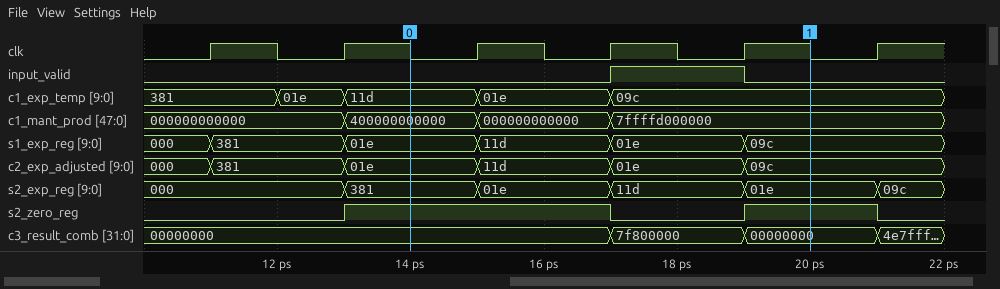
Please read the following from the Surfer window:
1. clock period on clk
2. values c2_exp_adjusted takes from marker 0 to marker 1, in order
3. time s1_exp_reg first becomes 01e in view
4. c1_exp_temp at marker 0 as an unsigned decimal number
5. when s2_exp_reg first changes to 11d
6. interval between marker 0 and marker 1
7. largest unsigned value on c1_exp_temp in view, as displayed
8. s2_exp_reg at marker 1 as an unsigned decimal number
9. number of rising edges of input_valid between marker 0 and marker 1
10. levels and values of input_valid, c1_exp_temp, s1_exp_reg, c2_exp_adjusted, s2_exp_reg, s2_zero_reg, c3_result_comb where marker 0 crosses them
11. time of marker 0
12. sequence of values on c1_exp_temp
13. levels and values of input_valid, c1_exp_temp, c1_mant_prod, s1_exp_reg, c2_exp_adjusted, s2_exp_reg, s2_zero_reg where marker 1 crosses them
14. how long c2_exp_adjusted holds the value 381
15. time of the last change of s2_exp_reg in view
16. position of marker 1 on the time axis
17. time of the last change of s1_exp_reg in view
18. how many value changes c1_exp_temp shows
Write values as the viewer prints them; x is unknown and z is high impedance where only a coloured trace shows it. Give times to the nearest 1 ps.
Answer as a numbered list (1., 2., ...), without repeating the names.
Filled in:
1. 2 ps
2. 01e, 11d, 01e, 09c
3. 13 ps
4. 285
5. 17 ps
6. 6 ps
7. 381
8. 30
9. 1
10. input_valid=0, c1_exp_temp=11d, s1_exp_reg=01e, c2_exp_adjusted=01e, s2_exp_reg=381, s2_zero_reg=1, c3_result_comb=00000000
11. 14 ps
12. 381, 01e, 11d, 01e, 09c
13. input_valid=0, c1_exp_temp=09c, c1_mant_prod=7ffffd000000, s1_exp_reg=09c, c2_exp_adjusted=09c, s2_exp_reg=01e, s2_zero_reg=1
14. 2 ps
15. 21 ps
16. 20 ps
17. 19 ps
18. 4
